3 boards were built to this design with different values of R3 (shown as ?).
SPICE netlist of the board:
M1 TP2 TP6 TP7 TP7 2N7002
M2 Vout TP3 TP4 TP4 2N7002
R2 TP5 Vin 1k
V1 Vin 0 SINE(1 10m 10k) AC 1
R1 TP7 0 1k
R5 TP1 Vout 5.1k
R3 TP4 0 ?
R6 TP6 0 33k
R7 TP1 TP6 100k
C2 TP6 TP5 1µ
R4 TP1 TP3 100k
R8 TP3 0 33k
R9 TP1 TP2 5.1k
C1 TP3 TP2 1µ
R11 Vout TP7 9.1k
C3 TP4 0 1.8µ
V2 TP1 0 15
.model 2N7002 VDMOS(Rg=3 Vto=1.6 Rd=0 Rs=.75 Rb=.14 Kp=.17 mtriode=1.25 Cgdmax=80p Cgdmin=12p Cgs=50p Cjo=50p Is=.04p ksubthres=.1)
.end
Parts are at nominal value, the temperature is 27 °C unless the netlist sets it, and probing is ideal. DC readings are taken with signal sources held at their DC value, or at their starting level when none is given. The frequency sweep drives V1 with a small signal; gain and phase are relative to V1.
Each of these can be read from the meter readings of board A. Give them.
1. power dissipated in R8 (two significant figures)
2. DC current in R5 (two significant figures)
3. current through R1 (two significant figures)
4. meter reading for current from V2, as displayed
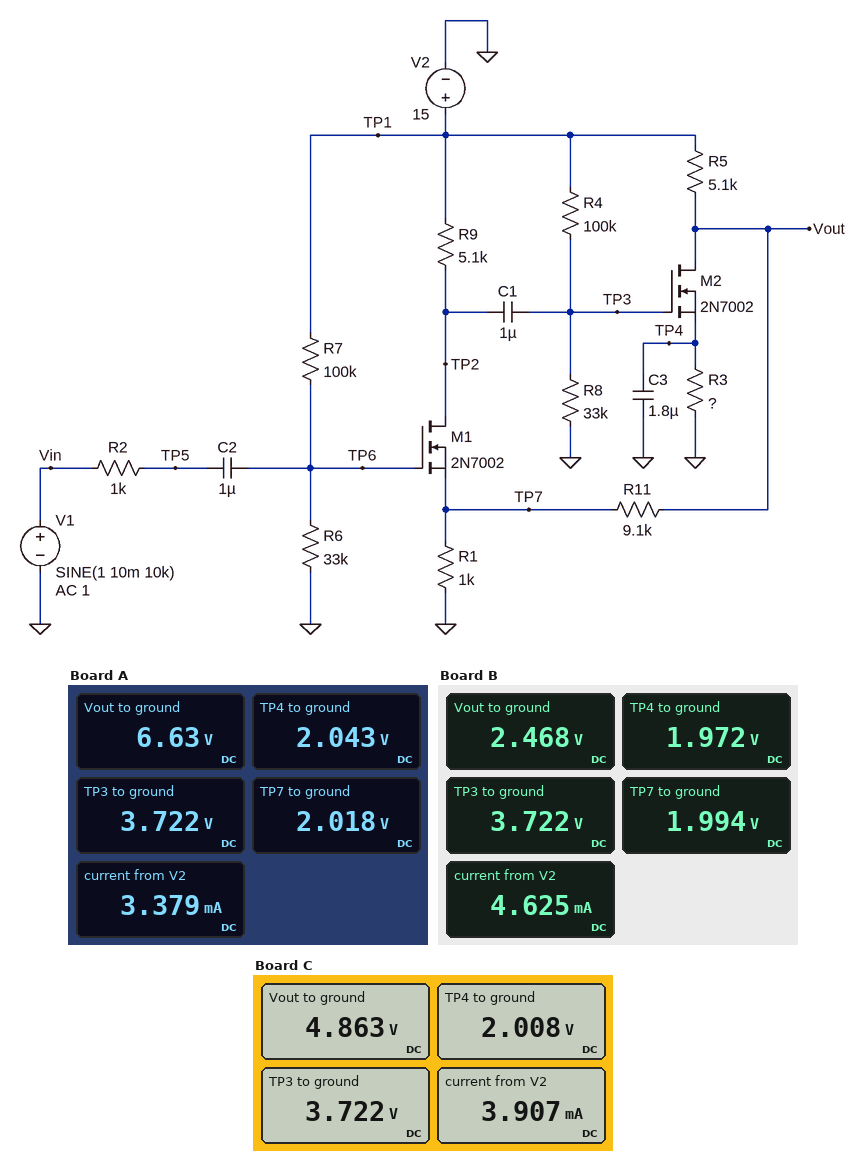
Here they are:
420 µW
1.6 mA
2.0 mA
3.379 mA
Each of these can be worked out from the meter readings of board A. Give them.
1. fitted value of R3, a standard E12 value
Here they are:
1.8 kΩ
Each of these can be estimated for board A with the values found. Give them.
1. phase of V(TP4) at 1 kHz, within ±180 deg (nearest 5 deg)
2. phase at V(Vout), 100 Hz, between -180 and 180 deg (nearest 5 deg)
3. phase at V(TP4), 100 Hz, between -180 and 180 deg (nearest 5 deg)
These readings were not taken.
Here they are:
95 deg
25 deg
140 deg
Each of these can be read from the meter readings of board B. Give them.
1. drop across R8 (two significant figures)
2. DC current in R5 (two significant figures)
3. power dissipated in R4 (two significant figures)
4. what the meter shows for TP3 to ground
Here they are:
3.7 V
2.5 mA
1.3 mW
3.722 V
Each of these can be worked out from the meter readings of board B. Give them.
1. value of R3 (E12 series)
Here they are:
820 Ω
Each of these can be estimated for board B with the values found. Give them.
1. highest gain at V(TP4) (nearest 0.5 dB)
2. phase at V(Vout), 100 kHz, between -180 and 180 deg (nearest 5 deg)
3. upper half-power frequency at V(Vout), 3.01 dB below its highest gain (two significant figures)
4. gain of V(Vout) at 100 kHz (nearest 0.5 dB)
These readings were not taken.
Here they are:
3.0 dB
-25 deg
220 kHz
18.5 dB
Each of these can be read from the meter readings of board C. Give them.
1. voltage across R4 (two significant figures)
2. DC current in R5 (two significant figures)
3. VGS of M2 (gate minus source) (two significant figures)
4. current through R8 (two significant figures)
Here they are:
11 V
2.0 mA
1.7 V
110 µA
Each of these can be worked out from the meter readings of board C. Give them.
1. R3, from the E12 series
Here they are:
1.2 kΩ
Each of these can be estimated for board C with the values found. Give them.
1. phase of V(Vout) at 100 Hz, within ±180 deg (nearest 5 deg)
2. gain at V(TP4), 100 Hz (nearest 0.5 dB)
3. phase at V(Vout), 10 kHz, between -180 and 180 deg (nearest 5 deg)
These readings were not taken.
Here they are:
20 deg
3.5 dB
0 deg
